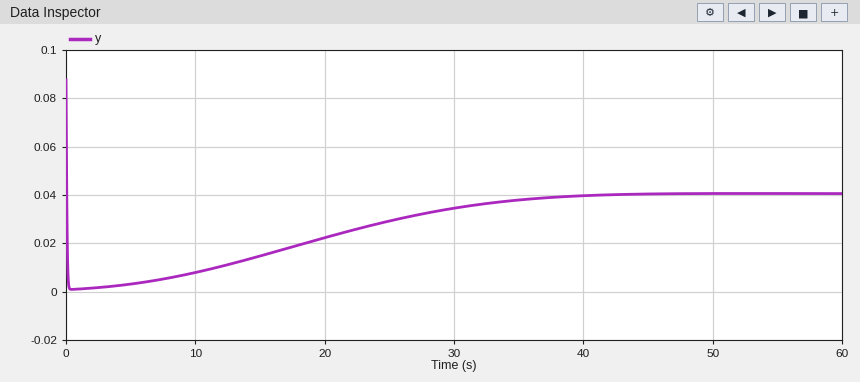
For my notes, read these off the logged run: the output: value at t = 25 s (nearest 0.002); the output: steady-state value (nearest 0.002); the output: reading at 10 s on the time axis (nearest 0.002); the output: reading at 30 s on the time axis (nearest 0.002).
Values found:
0.030
0.040
0.008
0.034
